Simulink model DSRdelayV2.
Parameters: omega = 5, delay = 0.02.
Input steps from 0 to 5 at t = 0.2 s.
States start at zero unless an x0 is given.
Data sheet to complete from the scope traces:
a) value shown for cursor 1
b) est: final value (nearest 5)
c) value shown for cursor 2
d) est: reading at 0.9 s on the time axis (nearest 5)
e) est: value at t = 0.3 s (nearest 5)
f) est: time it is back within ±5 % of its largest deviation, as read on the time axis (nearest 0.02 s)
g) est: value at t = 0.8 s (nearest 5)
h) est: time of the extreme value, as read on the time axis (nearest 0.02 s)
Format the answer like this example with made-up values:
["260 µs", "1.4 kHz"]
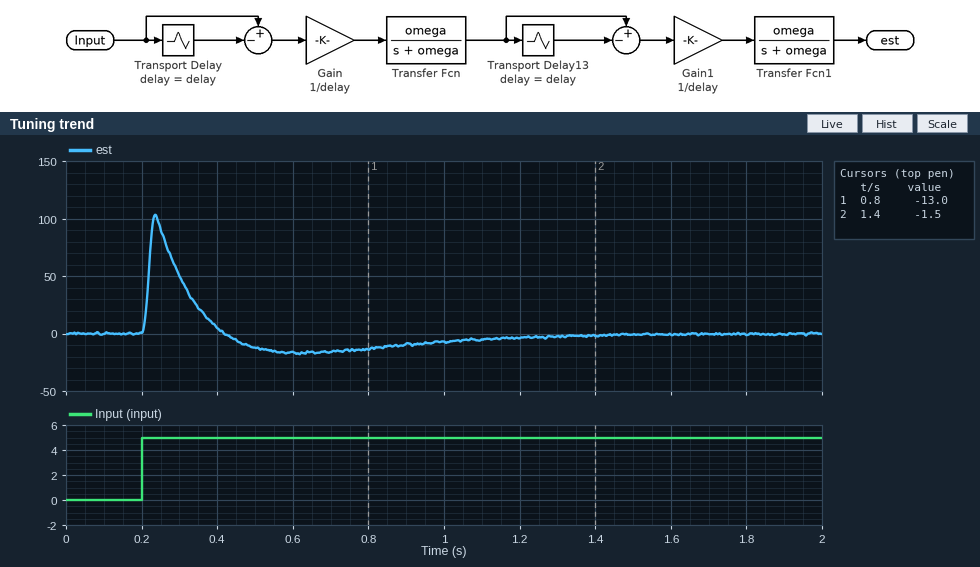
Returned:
["-13.0", "0", "-1.5", "-10", "50", "1.10 s", "-15", "0.24 s"]
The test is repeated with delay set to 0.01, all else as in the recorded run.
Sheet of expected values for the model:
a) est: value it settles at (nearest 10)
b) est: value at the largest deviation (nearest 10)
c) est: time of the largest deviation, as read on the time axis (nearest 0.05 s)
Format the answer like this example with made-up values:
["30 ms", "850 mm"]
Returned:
["0", "110", "0.20 s"]
